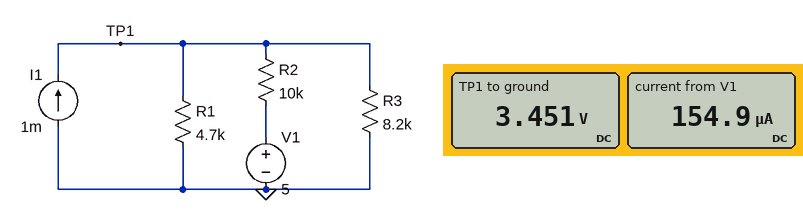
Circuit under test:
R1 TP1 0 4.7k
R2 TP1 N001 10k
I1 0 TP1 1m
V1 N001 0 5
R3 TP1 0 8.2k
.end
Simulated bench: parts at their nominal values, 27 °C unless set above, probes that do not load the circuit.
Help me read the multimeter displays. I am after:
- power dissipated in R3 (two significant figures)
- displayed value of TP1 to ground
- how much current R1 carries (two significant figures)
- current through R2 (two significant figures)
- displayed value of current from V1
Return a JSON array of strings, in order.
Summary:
["1.5 mW", "3.451 V", "730 µA", "150 µA", "154.9 µA"]
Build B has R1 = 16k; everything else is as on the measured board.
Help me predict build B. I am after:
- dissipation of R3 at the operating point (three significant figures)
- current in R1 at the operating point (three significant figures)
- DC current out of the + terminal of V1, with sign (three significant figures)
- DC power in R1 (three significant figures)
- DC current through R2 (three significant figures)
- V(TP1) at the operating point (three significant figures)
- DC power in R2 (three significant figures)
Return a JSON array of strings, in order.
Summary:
["3.39 mW", "330 µA", "-27.3 µA", "1.74 mW", "27.3 µA", "5.27 V", "7.47 µW"]
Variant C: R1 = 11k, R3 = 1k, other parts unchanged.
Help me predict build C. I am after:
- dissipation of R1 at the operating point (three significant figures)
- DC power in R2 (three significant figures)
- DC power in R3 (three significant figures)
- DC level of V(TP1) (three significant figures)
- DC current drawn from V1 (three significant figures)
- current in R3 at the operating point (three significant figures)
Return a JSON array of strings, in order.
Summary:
["144 µW", "1.40 mW", "1.59 mW", "1.26 V", "374 µA", "1.26 mA"]
